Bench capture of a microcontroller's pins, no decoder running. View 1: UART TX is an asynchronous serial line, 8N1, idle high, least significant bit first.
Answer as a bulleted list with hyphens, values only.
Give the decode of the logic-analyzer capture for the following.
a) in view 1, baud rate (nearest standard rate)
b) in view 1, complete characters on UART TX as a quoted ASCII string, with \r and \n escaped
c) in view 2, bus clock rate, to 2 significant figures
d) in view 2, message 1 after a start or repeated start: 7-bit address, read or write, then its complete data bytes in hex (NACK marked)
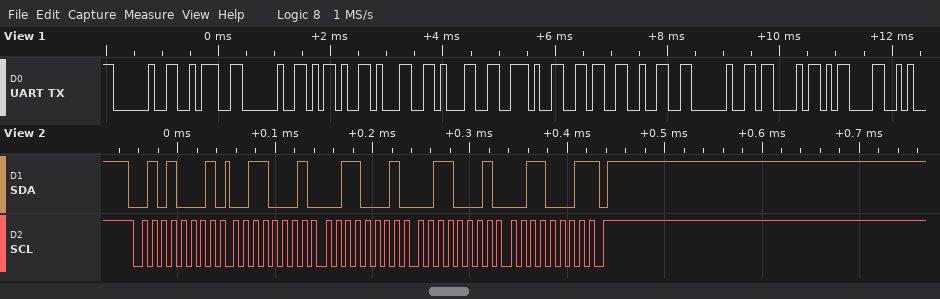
- 9600 baud
- " : -11.62 C\r"
- 100 kHz
- 0x28 read: 31 31 31 31 NACK
